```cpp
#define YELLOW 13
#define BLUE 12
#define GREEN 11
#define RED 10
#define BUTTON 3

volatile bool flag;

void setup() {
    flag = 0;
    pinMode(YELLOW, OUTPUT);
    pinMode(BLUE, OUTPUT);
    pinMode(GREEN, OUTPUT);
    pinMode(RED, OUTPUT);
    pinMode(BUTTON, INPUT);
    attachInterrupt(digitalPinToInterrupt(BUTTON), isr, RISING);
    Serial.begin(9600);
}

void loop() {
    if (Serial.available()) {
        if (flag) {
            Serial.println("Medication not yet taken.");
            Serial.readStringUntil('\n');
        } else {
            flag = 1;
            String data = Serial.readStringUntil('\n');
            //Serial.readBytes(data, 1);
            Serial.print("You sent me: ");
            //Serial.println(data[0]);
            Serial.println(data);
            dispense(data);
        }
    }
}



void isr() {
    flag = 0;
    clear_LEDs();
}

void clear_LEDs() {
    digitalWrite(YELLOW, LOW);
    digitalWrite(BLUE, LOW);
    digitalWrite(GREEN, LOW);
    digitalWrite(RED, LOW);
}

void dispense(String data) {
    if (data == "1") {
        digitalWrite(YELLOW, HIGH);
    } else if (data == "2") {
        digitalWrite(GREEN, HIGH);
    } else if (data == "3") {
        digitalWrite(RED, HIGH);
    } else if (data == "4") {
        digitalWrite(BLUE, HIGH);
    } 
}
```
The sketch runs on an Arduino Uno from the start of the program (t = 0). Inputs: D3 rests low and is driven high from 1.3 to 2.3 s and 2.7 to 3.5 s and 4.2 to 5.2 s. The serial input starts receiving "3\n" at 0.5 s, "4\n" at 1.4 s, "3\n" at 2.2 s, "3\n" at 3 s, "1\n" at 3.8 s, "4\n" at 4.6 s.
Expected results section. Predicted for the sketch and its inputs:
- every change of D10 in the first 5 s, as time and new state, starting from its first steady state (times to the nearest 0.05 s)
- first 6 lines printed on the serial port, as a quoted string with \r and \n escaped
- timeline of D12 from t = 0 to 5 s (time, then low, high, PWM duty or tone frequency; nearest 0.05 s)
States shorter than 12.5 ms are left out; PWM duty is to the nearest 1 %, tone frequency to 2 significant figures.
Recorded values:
0 s low; 0.5 s high; 1.3 s low; 3 s high; 4.2 s low
"You sent me: 3\r\nYou sent me: 4\r\nMedication not yet taken.\r\nYou sent me: 3\r\nMedication not yet taken.\r\nYou sent me: 4\r\n"
0 s low; 1.4 s high; 2.7 s low; 4.6 s high
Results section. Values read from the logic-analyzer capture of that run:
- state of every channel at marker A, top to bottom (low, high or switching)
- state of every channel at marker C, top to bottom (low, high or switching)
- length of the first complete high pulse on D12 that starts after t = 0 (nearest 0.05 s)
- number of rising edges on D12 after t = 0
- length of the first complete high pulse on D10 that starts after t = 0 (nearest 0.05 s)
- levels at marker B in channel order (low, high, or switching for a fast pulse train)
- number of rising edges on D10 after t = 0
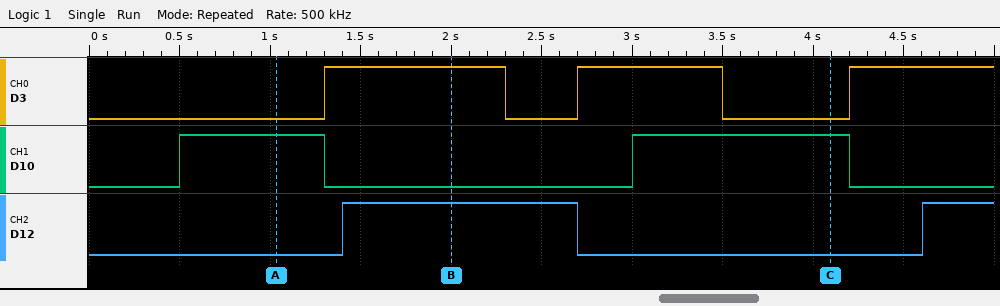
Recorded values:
D3 low, D10 high, D12 low
D3 low, D10 high, D12 low
1.30 s
2
0.80 s
D3 high, D10 low, D12 high
2
